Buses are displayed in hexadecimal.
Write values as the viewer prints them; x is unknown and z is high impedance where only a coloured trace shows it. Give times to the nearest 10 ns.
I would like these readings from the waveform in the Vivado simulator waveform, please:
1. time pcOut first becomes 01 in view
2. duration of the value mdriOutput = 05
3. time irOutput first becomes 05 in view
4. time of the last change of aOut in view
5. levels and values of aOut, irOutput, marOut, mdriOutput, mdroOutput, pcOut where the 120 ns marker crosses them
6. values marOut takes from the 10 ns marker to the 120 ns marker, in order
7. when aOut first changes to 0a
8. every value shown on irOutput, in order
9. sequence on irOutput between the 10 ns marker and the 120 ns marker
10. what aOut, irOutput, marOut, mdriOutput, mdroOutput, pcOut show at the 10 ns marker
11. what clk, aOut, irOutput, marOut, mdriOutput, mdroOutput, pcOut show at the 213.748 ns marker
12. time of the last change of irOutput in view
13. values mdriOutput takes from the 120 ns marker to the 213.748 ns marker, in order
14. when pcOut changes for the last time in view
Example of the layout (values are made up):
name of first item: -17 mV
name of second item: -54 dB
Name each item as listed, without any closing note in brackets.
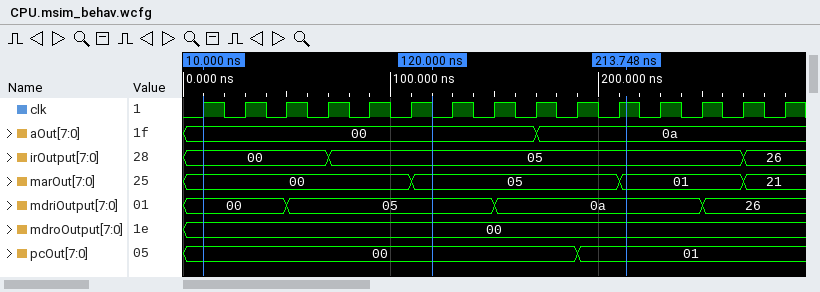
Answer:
time pcOut first becomes 01 in view: 190 ns
duration of the value mdriOutput = 05: 100 ns
time irOutput first becomes 05 in view: 70 ns
time of the last change of aOut in view: 170 ns
levels and values of aOut, irOutput, marOut, mdriOutput, mdroOutput, pcOut where the 120 ns marker crosses them: aOut=00, irOutput=05, marOut=05, mdriOutput=05, mdroOutput=00, pcOut=00
values marOut takes from the 10 ns marker to the 120 ns marker, in order: 00, 05
when aOut first changes to 0a: 170 ns
every value shown on irOutput, in order: 00, 05, 26
sequence on irOutput between the 10 ns marker and the 120 ns marker: 00, 05
what aOut, irOutput, marOut, mdriOutput, mdroOutput, pcOut show at the 10 ns marker: aOut=00, irOutput=00, marOut=00, mdriOutput=00, mdroOutput=00, pcOut=00
what clk, aOut, irOutput, marOut, mdriOutput, mdroOutput, pcOut show at the 213.748 ns marker: clk=1, aOut=0a, irOutput=05, marOut=01, mdriOutput=0a, mdroOutput=00, pcOut=01
time of the last change of irOutput in view: 270 ns
values mdriOutput takes from the 120 ns marker to the 213.748 ns marker, in order: 05, 0a
when pcOut changes for the last time in view: 190 ns
